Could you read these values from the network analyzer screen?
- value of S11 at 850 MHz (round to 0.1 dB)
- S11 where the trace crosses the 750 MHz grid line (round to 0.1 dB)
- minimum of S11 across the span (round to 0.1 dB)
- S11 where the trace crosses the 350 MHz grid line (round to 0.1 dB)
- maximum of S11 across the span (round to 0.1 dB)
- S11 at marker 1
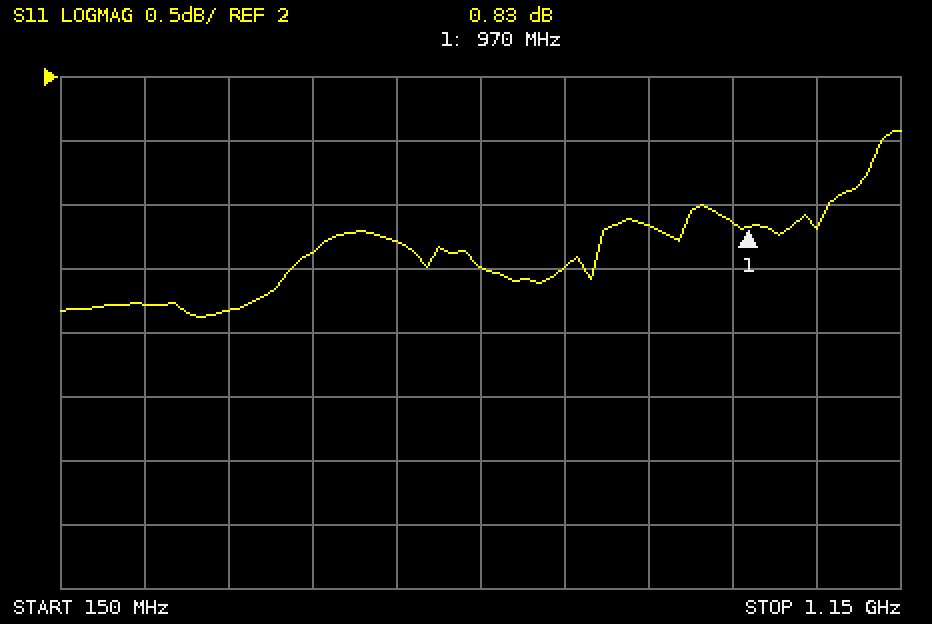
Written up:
0.8 dB
0.5 dB
0.1 dB
0.2 dB
1.6 dB
0.83 dB
